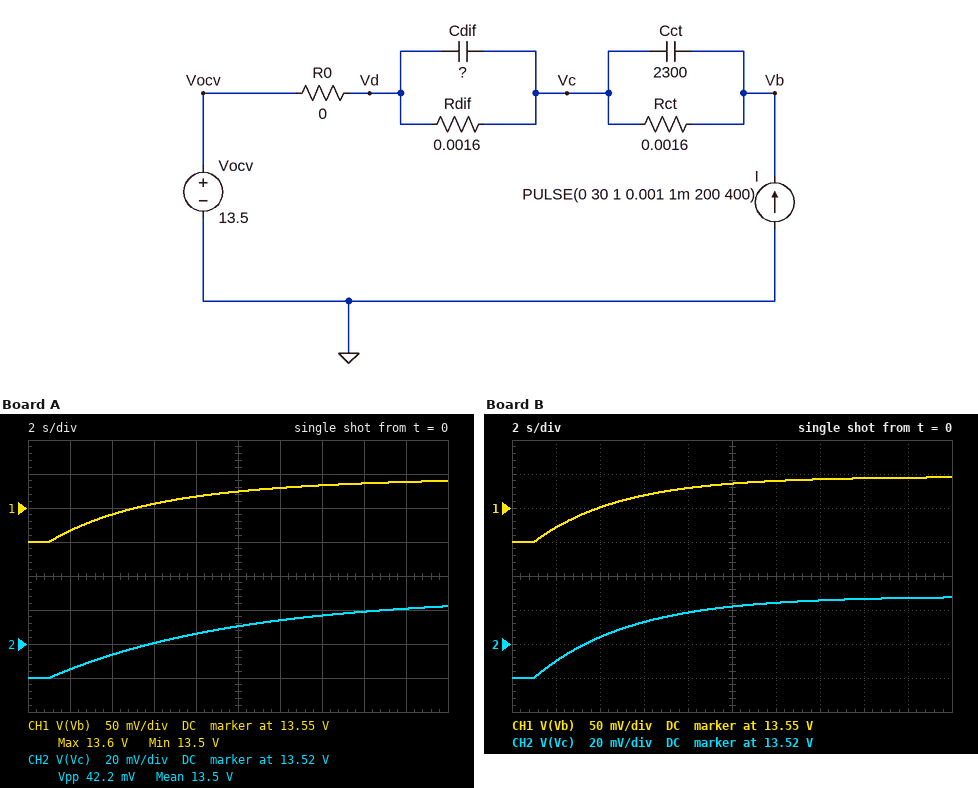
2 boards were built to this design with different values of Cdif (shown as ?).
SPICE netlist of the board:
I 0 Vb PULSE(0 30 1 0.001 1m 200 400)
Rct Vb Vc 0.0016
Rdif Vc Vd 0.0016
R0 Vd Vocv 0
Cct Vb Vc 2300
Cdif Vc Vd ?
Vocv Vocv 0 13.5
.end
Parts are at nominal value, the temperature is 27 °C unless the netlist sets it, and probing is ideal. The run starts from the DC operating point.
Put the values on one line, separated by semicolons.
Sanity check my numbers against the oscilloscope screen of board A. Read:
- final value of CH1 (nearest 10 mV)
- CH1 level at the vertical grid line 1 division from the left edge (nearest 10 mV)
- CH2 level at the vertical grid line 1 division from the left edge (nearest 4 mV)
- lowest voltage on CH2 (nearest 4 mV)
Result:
13.59 V; 13.52 V; 13.504 V; 13.500 V
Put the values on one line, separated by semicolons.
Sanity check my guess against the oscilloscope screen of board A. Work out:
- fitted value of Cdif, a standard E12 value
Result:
5.6 kF
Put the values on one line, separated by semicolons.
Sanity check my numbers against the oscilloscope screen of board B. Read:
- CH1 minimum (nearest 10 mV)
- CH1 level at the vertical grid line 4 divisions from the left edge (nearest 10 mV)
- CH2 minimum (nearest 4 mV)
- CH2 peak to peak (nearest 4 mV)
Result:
13.50 V; 13.58 V; 13.500 V; 48 mV
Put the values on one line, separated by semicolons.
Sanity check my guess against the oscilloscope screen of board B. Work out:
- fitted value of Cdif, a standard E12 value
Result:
2.7 kF
